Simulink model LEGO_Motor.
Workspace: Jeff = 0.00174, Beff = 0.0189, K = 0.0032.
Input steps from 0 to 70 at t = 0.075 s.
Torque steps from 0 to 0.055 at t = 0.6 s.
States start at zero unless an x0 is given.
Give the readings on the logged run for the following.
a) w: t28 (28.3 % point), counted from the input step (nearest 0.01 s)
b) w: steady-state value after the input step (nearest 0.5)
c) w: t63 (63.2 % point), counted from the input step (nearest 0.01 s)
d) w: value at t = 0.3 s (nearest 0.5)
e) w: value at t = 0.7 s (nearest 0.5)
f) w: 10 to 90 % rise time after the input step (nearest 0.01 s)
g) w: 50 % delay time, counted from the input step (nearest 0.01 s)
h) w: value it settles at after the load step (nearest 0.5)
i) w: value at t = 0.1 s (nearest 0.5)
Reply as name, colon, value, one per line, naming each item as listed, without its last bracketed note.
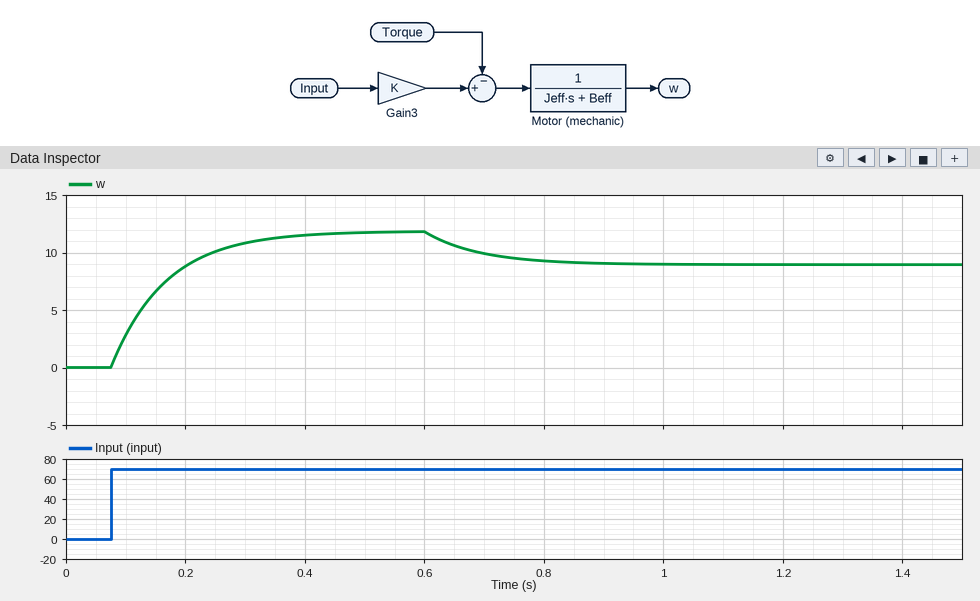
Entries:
w: t28 (28.3 % point), counted from the input step: 0.03 s
w: steady-state value after the input step: 12.0
w: t63 (63.2 % point), counted from the input step: 0.09 s
w: value at t = 0.3 s: 11.0
w: value at t = 0.7 s: 10.0
w: 10 to 90 % rise time after the input step: 0.20 s
w: 50 % delay time, counted from the input step: 0.06 s
w: value it settles at after the load step: 9.0
w: value at t = 0.1 s: 3.0
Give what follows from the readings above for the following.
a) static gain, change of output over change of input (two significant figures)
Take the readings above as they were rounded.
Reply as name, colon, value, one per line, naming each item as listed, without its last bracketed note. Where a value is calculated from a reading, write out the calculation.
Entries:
static gain, change of output over change of input: (12 - 0) / (70 - 0) = 0.17
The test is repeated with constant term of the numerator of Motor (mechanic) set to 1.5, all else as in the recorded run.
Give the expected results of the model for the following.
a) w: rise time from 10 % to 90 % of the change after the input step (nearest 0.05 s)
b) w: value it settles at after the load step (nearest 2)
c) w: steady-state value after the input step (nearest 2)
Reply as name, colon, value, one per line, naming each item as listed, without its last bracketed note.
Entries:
w: rise time from 10 % to 90 % of the change after the input step: 0.20 s
w: value it settles at after the load step: 14
w: steady-state value after the input step: 18
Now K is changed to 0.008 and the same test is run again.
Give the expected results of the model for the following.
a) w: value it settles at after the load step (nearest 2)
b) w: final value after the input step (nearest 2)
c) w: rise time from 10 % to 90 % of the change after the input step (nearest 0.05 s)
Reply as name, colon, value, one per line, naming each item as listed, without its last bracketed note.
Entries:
w: value it settles at after the load step: 26
w: final value after the input step: 30
w: rise time from 10 % to 90 % of the change after the input step: 0.20 s
